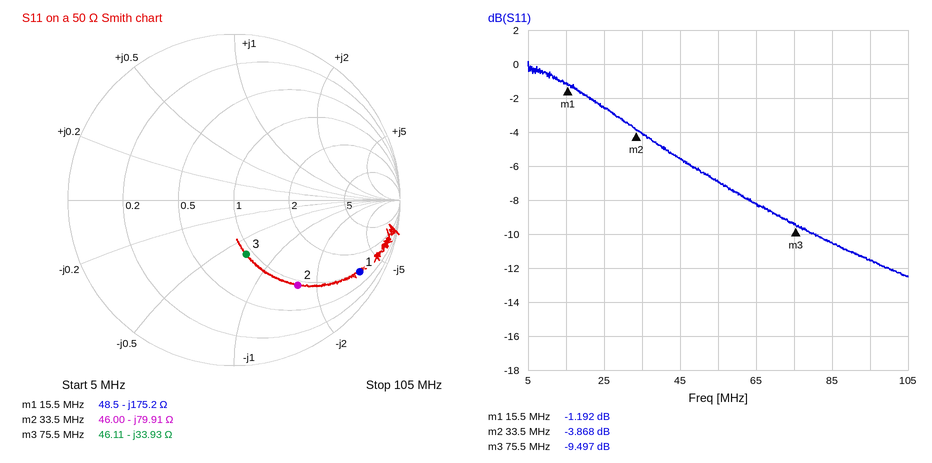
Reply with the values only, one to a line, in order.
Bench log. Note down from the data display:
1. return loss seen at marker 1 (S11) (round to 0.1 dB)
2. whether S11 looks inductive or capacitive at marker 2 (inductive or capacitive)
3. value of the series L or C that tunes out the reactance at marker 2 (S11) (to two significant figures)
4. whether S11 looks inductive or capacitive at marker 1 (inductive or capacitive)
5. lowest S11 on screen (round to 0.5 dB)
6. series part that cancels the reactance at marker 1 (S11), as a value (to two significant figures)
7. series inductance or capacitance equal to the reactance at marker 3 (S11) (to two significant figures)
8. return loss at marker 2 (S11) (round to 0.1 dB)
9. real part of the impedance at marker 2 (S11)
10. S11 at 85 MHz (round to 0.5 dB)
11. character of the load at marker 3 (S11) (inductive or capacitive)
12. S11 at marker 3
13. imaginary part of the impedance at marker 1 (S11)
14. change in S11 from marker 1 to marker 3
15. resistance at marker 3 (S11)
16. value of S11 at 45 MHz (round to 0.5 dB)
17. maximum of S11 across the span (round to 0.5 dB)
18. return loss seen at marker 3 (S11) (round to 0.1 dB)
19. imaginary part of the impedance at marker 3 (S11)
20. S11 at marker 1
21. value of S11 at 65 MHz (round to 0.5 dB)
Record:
1.2 dB
capacitive
380 nH
capacitive
-12.5 dB
1.8 µH
62 pF
3.9 dB
46.00 Ω
-10.5 dB
capacitive
-9.497 dB
-175.2 Ω
-8.305 dB
46.11 Ω
-5.5 dB
0.0 dB
9.5 dB
-33.93 Ω
-1.192 dB
-8.0 dB
